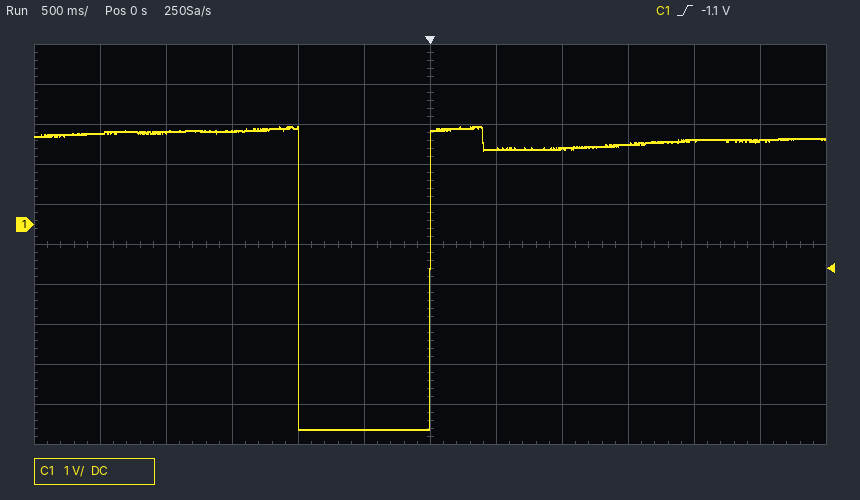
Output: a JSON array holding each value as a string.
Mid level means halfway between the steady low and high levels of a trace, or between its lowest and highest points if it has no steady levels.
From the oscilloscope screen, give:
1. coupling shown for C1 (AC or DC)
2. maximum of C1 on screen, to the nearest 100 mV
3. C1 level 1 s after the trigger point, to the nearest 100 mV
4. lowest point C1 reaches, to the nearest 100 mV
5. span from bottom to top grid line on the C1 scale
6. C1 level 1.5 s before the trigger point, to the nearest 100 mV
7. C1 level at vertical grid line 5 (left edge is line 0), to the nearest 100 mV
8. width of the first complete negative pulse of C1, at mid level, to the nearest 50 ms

["DC", "2.4 V", "1.9 V", "-5.1 V", "10 V", "2.3 V", "-5.1 V", "1.00 s"]
